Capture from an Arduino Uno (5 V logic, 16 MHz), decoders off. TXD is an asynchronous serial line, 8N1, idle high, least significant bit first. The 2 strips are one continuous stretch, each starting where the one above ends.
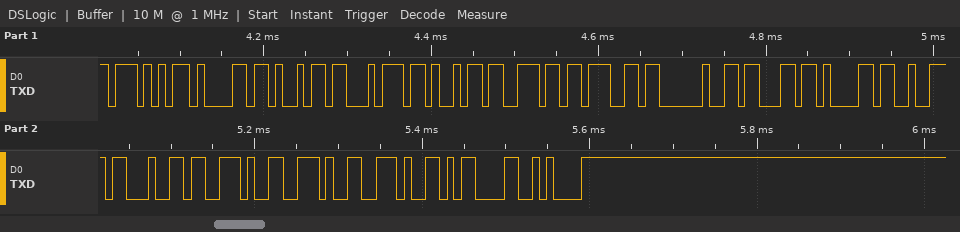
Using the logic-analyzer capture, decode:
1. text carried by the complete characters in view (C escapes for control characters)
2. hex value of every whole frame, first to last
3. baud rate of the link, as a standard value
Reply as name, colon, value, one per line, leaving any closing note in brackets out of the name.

text carried by the complete characters in view: "Waiting card...\r\n"
hex value of every whole frame, first to last: 0x57 0x61 0x69 0x74 0x69 0x6E 0x67 0x20 0x63 0x61 0x72 0x64 0x2E 0x2E 0x2E 0x0D 0x0A
baud rate of the link, as a standard value: 115200 baud
